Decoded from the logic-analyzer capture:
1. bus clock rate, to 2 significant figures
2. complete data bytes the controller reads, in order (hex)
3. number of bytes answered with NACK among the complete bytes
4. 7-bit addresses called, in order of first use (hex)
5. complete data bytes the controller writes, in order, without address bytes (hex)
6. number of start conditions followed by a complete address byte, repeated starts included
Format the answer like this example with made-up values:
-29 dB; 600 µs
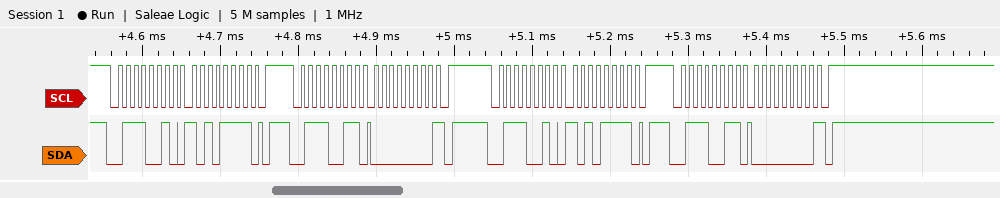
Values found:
100 kHz; 00 00; 2; 0x39; AF AF; 4
